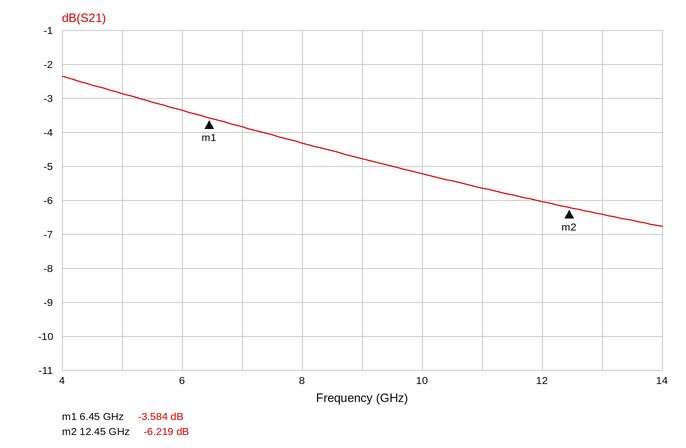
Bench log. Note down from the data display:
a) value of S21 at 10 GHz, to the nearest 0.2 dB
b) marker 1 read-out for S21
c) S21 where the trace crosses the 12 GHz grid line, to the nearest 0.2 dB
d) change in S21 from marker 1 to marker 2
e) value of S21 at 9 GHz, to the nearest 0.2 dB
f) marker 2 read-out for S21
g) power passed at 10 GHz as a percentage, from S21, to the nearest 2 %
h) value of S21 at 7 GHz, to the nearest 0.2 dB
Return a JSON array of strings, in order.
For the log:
["-5.2 dB", "-3.584 dB", "-6.0 dB", "-2.635 dB", "-4.8 dB", "-6.219 dB", "30 %", "-3.8 dB"]
